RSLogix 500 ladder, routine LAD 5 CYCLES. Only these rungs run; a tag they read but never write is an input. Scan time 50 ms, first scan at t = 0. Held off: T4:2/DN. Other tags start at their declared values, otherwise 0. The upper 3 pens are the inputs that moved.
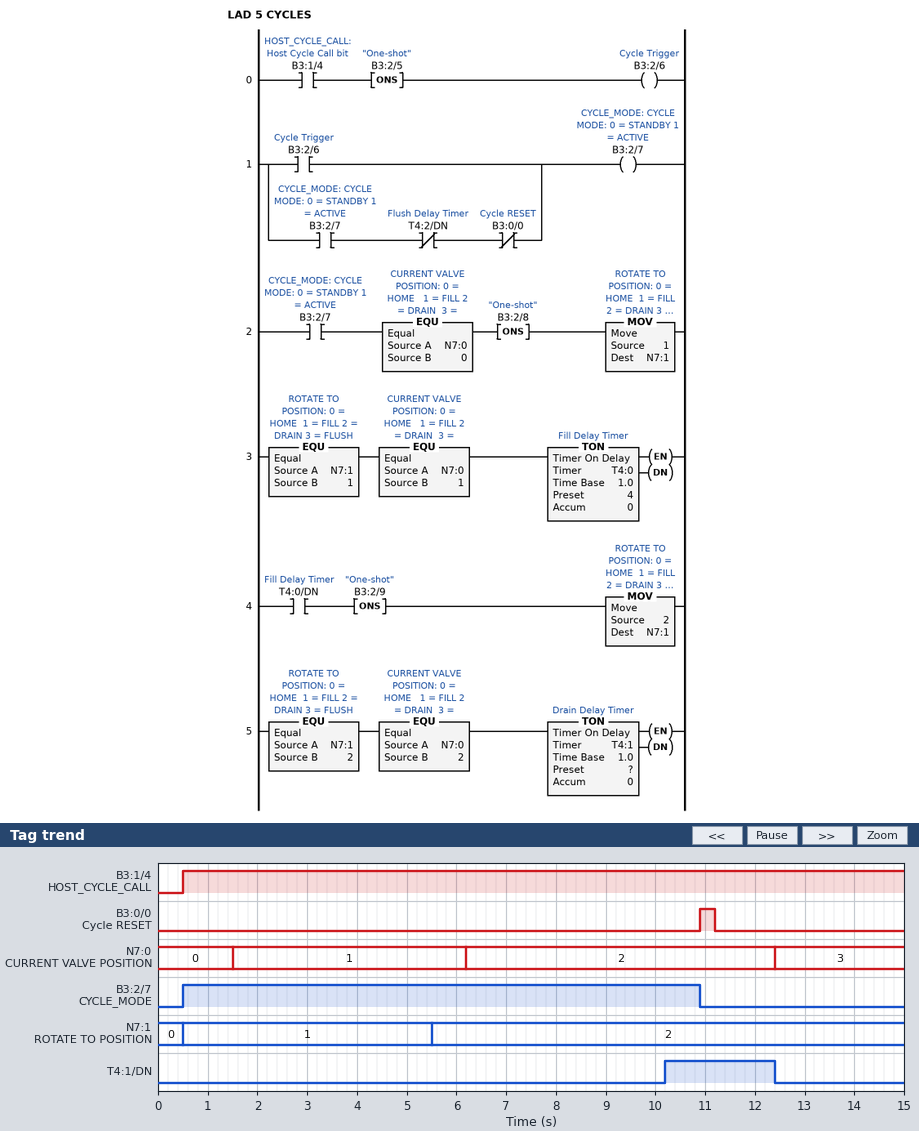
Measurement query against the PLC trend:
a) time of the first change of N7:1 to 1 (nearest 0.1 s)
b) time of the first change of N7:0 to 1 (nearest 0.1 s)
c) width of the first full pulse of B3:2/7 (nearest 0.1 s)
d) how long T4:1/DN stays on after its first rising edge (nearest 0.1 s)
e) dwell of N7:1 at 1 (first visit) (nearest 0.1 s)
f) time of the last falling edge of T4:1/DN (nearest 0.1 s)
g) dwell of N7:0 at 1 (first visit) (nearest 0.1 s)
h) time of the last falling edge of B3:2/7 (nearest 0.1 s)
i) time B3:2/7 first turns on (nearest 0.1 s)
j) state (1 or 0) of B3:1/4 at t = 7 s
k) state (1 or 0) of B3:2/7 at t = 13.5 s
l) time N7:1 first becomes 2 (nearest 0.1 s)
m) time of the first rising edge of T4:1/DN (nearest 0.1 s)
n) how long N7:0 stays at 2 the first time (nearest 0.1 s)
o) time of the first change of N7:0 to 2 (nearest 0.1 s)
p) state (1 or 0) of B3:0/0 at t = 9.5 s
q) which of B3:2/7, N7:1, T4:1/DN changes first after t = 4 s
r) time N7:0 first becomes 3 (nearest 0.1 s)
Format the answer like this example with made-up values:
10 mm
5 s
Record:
0.5 s
1.5 s
10.4 s
2.2 s
5.0 s
12.4 s
4.7 s
10.9 s
0.5 s
1
0
5.5 s
10.2 s
6.2 s
6.2 s
0
N7:1
12.4 s
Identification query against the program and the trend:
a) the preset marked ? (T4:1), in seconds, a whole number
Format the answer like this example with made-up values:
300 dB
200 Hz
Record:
4 s
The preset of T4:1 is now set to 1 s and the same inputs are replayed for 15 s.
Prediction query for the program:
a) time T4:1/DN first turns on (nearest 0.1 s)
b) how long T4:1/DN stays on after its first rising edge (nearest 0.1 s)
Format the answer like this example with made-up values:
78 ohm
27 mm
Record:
7.2 s
5.2 s
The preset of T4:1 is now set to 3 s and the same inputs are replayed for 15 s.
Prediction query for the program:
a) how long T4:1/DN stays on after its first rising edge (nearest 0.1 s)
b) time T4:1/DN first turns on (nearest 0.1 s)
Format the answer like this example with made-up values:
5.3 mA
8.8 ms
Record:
3.2 s
9.2 s
